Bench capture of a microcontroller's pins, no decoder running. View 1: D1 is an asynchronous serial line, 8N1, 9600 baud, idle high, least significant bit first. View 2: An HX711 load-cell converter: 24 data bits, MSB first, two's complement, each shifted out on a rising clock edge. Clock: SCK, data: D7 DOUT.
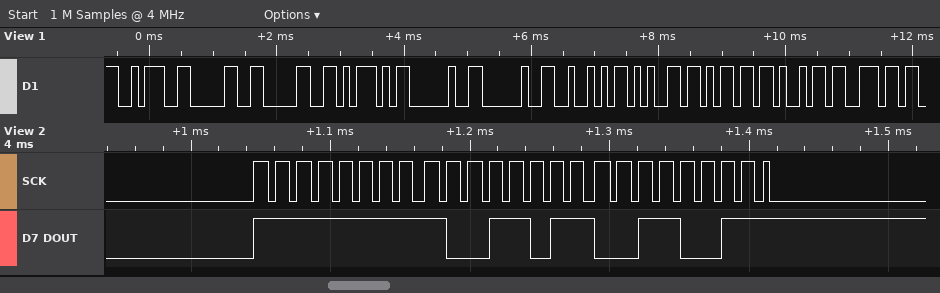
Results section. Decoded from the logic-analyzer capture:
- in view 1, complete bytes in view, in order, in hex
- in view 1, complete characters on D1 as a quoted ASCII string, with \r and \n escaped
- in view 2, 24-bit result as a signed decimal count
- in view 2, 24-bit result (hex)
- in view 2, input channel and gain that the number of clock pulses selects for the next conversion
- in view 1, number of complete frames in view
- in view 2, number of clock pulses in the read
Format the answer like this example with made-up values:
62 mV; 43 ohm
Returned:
3A 30 30 5D 20 20 52 65 6D 69 6E; ":00]  Remin"; -25805; 0xFF9B33; channel A, gain 128; 11; 25
